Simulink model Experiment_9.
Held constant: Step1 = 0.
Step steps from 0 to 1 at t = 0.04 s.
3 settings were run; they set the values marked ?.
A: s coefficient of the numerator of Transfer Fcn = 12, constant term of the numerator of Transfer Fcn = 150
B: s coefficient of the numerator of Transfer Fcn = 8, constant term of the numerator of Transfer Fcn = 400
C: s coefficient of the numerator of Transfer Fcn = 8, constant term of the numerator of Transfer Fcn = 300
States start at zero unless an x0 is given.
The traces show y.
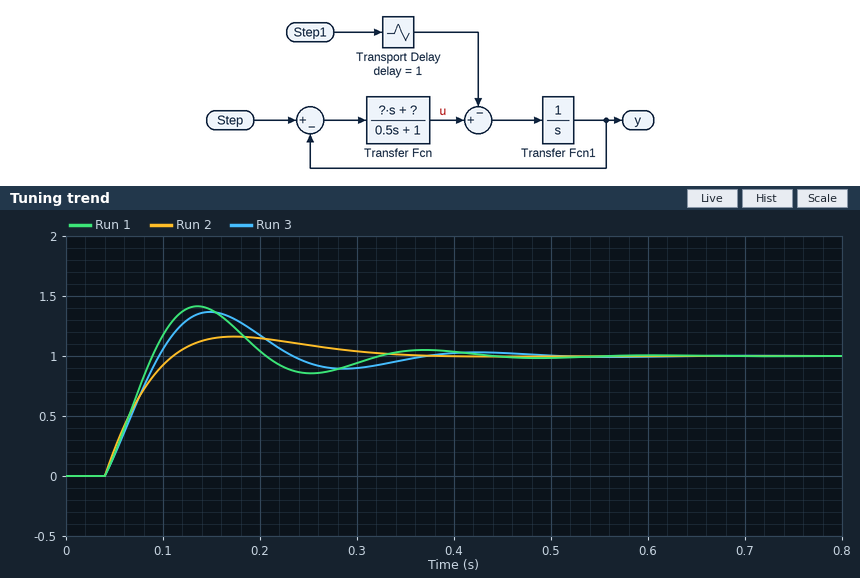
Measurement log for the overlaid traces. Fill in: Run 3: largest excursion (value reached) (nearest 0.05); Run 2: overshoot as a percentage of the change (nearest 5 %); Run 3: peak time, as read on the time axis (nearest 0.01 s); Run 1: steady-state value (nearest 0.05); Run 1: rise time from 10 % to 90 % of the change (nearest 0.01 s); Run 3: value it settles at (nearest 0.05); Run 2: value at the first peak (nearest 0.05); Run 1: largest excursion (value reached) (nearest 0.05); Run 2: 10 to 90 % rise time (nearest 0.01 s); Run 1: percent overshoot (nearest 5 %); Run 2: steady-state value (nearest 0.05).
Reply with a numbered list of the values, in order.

1. 1.35
2. 15 %
3. 0.15 s
4. 1.00
5. 0.04 s
6. 1.00
7. 1.15
8. 1.40
9. 0.05 s
10. 40 %
11. 1.00
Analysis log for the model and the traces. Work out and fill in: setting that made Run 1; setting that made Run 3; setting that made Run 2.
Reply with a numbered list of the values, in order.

1. B
2. C
3. A
